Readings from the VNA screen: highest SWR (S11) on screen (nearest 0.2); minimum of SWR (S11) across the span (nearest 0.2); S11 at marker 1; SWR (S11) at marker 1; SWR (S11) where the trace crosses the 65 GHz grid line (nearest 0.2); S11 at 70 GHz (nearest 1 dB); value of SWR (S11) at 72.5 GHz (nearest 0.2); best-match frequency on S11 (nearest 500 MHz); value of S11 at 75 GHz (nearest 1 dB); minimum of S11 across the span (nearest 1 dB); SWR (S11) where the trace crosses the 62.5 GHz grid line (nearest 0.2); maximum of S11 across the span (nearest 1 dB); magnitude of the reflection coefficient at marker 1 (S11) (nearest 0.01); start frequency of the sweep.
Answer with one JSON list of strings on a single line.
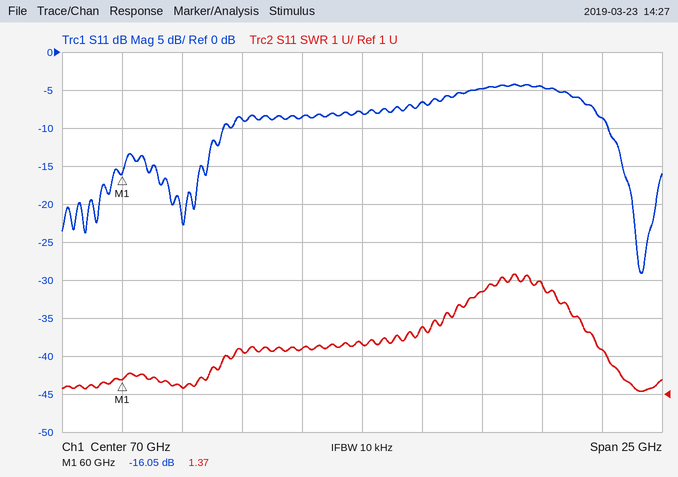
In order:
["4.2", "1.0", "-16.05 dB", "1.37", "2.2", "-8 dB", "2.8", "81.5 GHz", "-5 dB", "-29 dB", "1.2", "-4 dB", "0.16", "57.5 GHz"]
